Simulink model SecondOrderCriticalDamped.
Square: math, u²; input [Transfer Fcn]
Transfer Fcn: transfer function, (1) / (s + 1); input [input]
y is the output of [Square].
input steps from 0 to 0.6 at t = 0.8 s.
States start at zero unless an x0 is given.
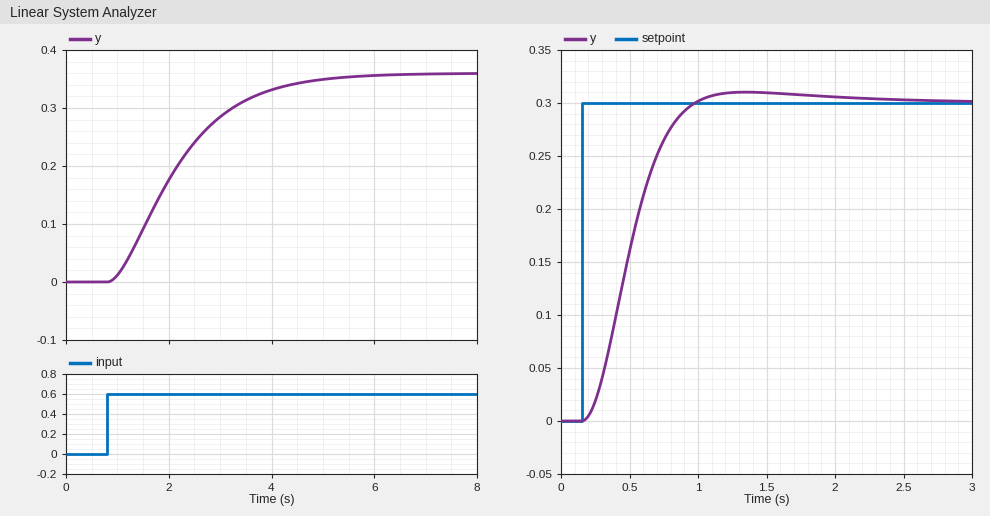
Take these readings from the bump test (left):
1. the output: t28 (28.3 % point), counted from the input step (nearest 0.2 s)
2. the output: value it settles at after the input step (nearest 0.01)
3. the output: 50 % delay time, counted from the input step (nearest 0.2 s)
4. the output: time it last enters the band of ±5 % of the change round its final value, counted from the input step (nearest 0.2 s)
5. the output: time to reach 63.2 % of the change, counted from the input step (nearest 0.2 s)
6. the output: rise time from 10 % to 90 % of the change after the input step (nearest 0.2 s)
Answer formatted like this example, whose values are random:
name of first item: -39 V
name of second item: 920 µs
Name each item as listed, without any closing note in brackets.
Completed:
the output: t28 (28.3 % point), counted from the input step: 0.8 s
the output: value it settles at after the input step: 0.36
the output: 50 % delay time, counted from the input step: 1.2 s
the output: time it last enters the band of ±5 % of the change round its final value, counted from the input step: 3.6 s
the output: time to reach 63.2 % of the change, counted from the input step: 1.6 s
the output: rise time from 10 % to 90 % of the change after the input step: 2.6 s
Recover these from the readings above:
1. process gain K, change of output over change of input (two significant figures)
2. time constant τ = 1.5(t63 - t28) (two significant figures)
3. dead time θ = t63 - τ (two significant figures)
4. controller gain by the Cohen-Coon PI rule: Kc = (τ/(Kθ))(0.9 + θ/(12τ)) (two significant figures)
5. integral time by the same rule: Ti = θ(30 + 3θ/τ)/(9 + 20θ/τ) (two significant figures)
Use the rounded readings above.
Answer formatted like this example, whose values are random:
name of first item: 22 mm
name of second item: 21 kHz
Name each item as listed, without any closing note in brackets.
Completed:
process gain K, change of output over change of input: 0.60
time constant τ = 1.5(t63 - t28): 1.2 s
dead time θ = t63 - τ: 0.40 s
controller gain by the Cohen-Coon PI rule: Kc = (τ/(Kθ))(0.9 + θ/(12τ)): 4.6
integral time by the same rule: Ti = θ(30 + 3θ/τ)/(9 + 20θ/τ): 0.79 s
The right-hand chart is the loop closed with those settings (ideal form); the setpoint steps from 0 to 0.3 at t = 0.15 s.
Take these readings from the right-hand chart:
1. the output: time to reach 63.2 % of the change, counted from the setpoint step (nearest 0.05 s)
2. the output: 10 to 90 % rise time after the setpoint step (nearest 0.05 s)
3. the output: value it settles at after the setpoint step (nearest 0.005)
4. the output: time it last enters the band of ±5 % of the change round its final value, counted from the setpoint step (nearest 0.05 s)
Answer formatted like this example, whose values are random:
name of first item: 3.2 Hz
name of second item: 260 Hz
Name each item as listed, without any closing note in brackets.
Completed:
the output: time to reach 63.2 % of the change, counted from the setpoint step: 0.40 s
the output: 10 to 90 % rise time after the setpoint step: 0.50 s
the output: value it settles at after the setpoint step: 0.300
the output: time it last enters the band of ±5 % of the change round its final value, counted from the setpoint step: 0.70 s
